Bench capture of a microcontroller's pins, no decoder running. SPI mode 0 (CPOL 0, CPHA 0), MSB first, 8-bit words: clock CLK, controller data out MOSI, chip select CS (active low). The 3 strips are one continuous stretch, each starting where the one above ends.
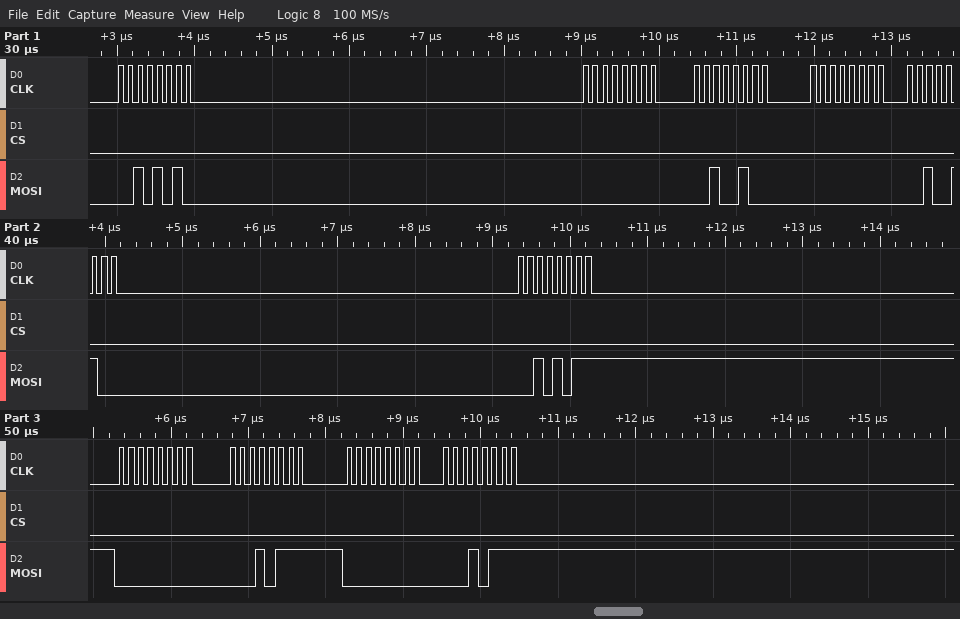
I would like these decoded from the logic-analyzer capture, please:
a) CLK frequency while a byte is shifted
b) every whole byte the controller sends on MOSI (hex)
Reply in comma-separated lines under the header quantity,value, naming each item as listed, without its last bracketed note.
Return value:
quantity,value
CLK frequency while a byte is shifted,8 MHz
every whole byte the controller sends on MOSI,2A 00 24 00 24 2B 00 17 00 17
